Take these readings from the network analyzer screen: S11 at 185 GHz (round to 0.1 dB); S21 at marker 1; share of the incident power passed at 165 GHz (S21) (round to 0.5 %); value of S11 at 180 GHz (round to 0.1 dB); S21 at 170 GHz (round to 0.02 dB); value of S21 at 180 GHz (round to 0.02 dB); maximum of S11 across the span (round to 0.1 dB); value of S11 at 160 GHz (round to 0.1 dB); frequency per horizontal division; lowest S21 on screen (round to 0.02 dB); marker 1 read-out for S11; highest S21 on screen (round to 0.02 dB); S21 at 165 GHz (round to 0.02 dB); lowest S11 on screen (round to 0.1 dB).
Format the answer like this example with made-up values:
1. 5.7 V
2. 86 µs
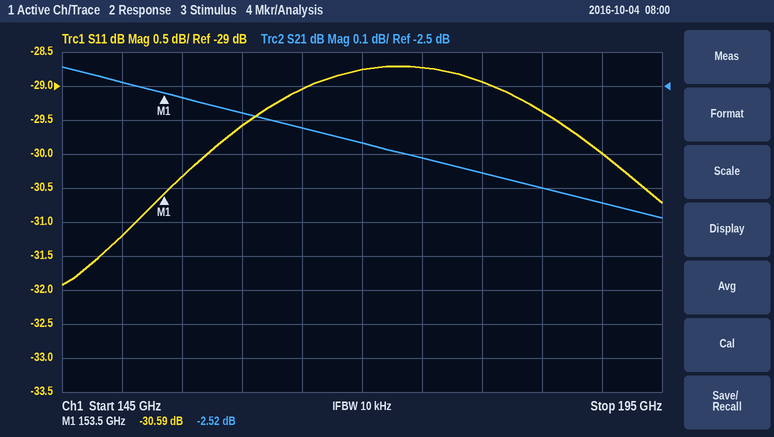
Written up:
1. -29.4 dB
2. -2.52 dB
3. 54.5 %
4. -28.9 dB
5. -2.66 dB
6. -2.76 dB
7. -28.7 dB
8. -29.6 dB
9. 5 GHz
10. -2.88 dB
11. -30.59 dB
12. -2.44 dB
13. -2.62 dB
14. -31.9 dB
